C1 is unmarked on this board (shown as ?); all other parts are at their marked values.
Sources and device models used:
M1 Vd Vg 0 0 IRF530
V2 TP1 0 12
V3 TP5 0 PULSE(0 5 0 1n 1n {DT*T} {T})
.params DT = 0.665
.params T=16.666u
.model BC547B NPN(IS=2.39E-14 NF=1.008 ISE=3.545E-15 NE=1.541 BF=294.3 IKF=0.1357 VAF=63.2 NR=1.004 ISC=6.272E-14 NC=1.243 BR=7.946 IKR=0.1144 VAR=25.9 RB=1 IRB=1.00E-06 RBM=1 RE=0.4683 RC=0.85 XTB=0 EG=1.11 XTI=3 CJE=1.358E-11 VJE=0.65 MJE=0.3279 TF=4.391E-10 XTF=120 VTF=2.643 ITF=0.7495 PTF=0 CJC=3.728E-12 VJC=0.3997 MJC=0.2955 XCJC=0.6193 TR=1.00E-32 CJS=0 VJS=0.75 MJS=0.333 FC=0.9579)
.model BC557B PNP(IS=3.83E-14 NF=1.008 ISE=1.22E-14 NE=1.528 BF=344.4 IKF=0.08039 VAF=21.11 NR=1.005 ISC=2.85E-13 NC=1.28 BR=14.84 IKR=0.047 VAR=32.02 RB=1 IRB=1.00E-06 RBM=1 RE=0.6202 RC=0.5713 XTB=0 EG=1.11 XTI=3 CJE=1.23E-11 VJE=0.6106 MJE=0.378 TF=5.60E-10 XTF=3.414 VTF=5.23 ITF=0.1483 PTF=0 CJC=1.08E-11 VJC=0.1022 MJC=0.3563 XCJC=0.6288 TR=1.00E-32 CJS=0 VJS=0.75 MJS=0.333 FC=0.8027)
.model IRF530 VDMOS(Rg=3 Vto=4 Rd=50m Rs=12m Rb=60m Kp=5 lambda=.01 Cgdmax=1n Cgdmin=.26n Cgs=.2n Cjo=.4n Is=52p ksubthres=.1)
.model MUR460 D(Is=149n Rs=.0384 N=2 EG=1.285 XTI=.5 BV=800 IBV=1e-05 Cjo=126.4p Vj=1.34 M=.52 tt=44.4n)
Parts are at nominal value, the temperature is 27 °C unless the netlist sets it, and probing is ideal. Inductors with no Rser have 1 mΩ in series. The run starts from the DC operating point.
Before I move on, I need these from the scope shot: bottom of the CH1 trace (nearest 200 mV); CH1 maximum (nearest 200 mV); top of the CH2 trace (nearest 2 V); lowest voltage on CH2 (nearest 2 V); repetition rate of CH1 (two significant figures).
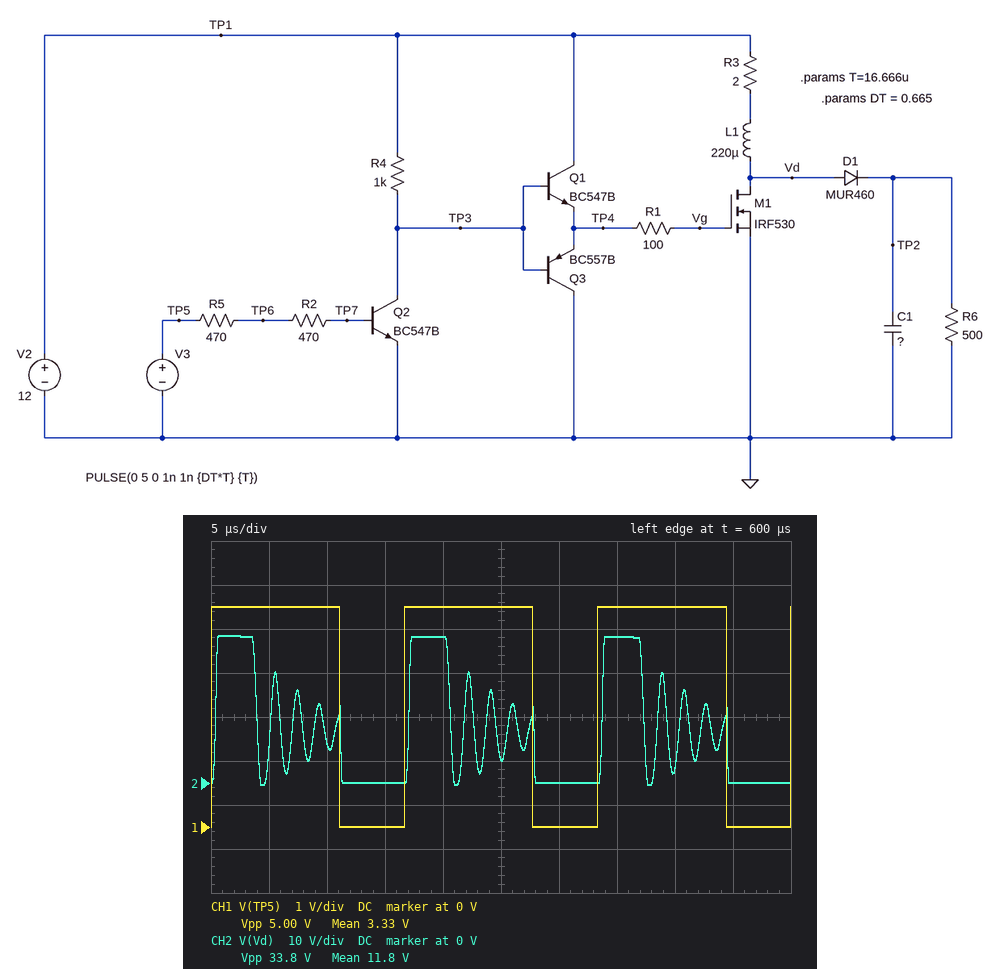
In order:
0 V
5.0 V
34 V
0 V
60 kHz
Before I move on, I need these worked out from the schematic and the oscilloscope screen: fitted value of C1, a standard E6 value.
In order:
6.8 µF
